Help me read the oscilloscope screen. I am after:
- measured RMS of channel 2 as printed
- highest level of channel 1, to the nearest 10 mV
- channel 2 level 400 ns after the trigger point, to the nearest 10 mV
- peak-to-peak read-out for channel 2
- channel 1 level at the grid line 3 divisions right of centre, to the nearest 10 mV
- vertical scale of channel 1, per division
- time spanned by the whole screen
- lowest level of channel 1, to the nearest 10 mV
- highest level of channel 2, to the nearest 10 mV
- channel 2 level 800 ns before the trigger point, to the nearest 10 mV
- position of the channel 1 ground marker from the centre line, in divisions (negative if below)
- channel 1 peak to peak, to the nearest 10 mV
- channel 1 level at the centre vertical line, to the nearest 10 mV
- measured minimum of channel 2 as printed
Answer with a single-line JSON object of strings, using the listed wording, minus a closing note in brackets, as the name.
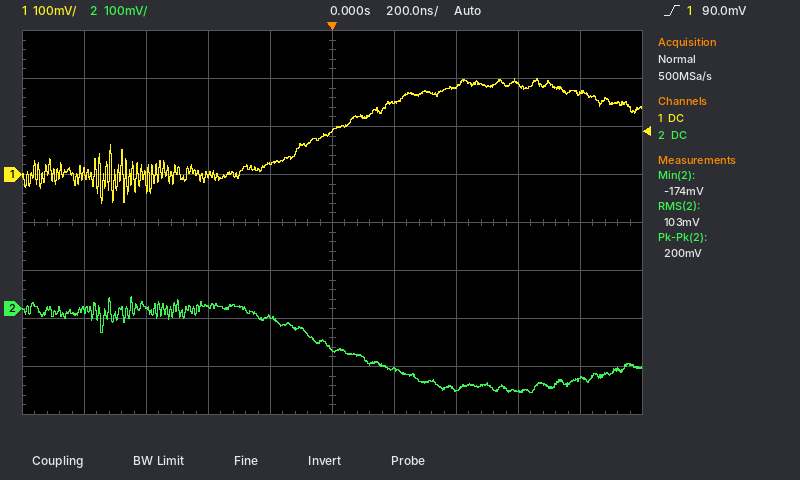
{"measured RMS of channel 2 as printed": "103 mV", "highest level of channel 1, to the nearest 10 mV": "200 mV", "channel 2 level 400 ns after the trigger point, to the nearest 10 mV": "-170 mV", "peak-to-peak read-out for channel 2": "200 mV", "channel 1 level at the grid line 3 divisions right of centre, to the nearest 10 mV": "190 mV", "vertical scale of channel 1, per division": "100 mV", "time spanned by the whole screen": "2 µs", "lowest level of channel 1, to the nearest 10 mV": "-60 mV", "highest level of channel 2, to the nearest 10 mV": "30 mV", "channel 2 level 800 ns before the trigger point, to the nearest 10 mV": "0 mV", "position of the channel 1 ground marker from the centre line, in divisions": "+1.0 div", "channel 1 peak to peak, to the nearest 10 mV": "260 mV", "channel 1 level at the centre vertical line, to the nearest 10 mV": "90 mV", "measured minimum of channel 2 as printed": "-174 mV"}
